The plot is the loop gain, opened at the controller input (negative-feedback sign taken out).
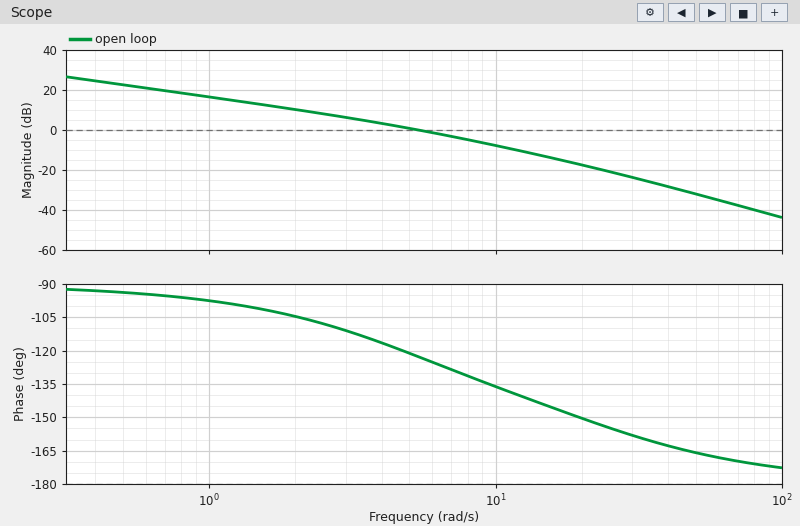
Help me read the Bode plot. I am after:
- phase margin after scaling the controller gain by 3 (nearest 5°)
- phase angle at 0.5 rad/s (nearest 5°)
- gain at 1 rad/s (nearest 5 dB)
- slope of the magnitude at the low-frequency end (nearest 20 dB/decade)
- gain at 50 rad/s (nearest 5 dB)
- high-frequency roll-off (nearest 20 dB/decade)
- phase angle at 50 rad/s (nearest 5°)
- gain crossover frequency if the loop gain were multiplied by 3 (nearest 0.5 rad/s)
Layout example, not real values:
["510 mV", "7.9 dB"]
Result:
["40°", "-95°", "15 dB", "-20 dB/decade", "-30 dB", "-40 dB/decade", "-165°", "11.5 rad/s"]
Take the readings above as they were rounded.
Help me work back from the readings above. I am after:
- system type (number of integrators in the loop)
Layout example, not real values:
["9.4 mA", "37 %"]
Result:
["1"]
